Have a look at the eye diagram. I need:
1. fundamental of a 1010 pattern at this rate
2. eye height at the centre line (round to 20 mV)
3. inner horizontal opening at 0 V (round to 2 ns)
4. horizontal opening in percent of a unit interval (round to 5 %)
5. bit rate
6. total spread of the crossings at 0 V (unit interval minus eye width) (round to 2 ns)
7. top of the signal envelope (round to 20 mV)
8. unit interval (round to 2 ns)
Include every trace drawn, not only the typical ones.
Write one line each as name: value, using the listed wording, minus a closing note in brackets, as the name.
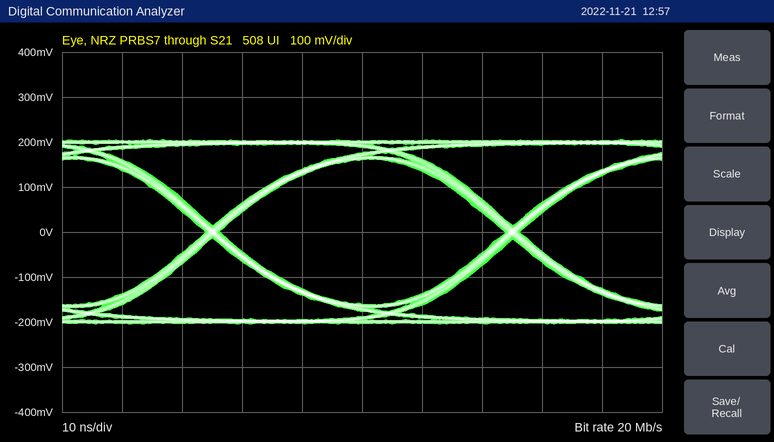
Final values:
fundamental of a 1010 pattern at this rate: 10 MHz
eye height at the centre line: 320 mV
inner horizontal opening at 0 V: 48 ns
horizontal opening in percent of a unit interval: 95 %
bit rate: 20 Mb/s
total spread of the crossings at 0 V (unit interval minus eye width): 2 ns
top of the signal envelope: 200 mV
unit interval: 50 ns
